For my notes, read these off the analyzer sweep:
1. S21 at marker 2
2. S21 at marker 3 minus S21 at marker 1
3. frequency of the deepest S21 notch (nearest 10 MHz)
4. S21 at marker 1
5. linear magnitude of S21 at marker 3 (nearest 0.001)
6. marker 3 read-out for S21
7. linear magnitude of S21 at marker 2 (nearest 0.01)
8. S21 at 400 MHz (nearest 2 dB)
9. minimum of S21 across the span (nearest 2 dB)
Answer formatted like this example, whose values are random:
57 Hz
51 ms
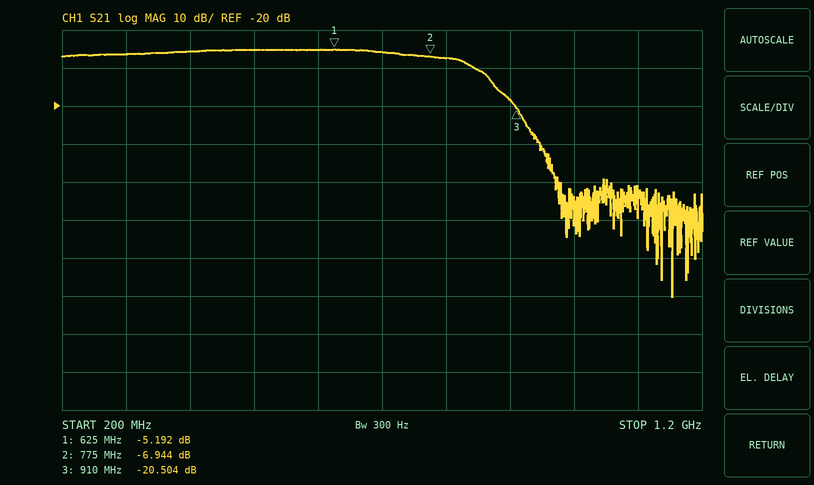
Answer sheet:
-6.944 dB
-15.312 dB
1.15 GHz
-5.192 dB
0.094
-20.504 dB
0.45
-6 dB
-70 dB
